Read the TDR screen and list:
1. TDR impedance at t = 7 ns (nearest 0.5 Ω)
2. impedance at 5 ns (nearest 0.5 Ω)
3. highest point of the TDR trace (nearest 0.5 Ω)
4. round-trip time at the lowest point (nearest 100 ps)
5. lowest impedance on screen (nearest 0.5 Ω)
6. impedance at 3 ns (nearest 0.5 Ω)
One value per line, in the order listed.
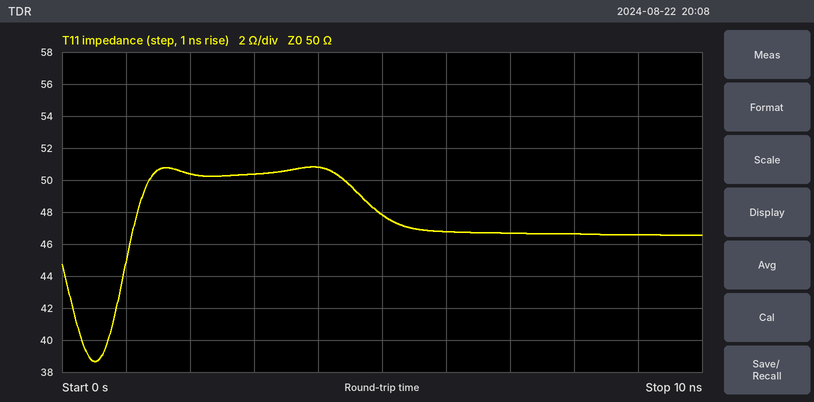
46.5 Ω
48.0 Ω
51.0 Ω
500 ps
38.5 Ω
50.5 Ω
